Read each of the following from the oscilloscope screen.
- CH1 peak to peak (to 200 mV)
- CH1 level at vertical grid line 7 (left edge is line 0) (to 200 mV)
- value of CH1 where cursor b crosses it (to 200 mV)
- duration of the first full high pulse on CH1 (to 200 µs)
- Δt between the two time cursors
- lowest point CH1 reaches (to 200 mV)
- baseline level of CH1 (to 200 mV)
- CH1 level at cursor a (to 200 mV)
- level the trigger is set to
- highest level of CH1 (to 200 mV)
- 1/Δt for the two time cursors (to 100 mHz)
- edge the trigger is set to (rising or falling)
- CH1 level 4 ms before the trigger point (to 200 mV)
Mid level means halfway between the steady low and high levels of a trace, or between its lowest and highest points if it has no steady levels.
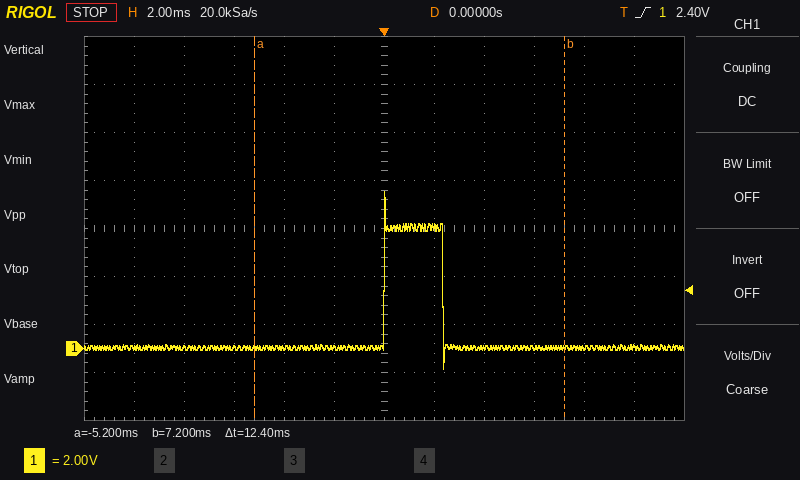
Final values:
7.4 V
5.0 V
0.0 V
2.4 ms
12.4 ms
-800 mV
0.0 V
0.0 V
2.40 V
6.6 V
80.6 Hz
rising
0.0 V
